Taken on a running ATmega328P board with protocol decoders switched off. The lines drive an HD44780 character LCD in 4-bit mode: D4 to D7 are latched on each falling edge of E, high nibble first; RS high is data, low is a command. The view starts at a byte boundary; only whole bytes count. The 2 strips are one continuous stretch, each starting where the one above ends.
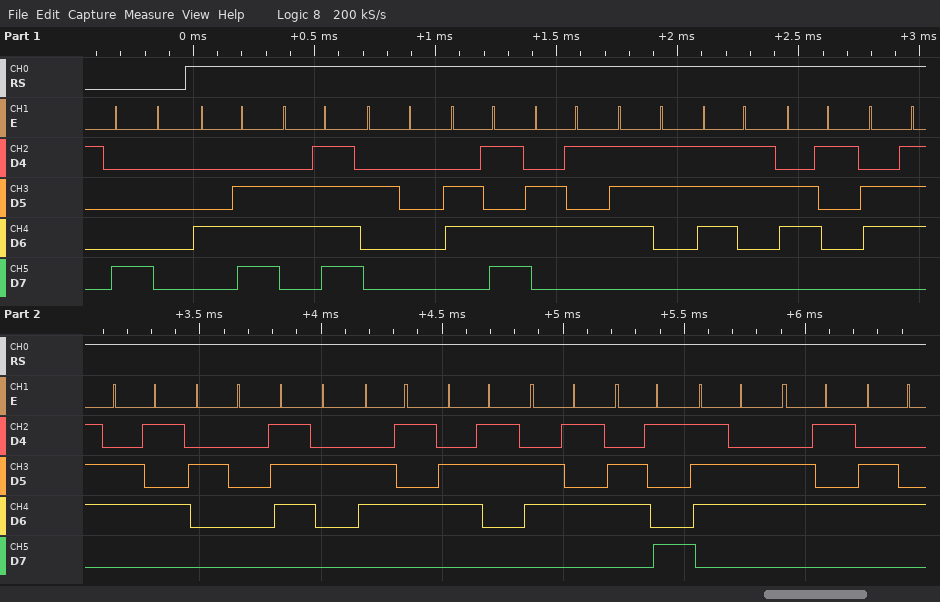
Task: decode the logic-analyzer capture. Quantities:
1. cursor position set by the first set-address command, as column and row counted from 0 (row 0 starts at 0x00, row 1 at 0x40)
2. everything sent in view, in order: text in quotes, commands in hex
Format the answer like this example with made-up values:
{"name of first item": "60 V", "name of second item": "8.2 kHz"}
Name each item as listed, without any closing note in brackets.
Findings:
{"cursor position set by the first set-address command, as column and row counted from 0": "column 0, row 0", "everything sent in view, in order: text in quotes, commands in hex": "0x80 \"No message received\""}
